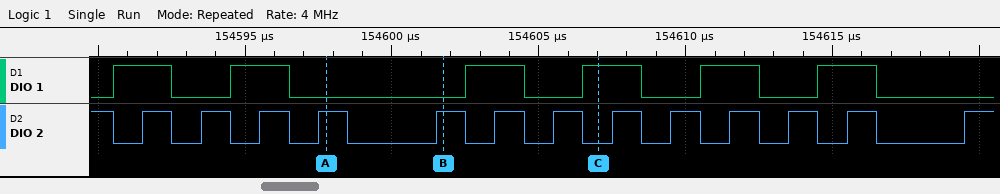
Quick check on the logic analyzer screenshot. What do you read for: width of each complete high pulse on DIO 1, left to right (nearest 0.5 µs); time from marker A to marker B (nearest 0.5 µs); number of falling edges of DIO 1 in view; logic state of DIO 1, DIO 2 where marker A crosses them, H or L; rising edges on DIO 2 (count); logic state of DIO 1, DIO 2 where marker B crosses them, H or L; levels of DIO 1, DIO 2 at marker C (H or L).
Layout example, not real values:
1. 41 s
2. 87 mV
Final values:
1. 2 µs, 2 µs, 2 µs, 2 µs, 2 µs, 2 µs
2. 4 µs
3. 6
4. DIO 1=L, DIO 2=H
5. 13
6. DIO 1=L, DIO 2=H
7. DIO 1=H, DIO 2=L
